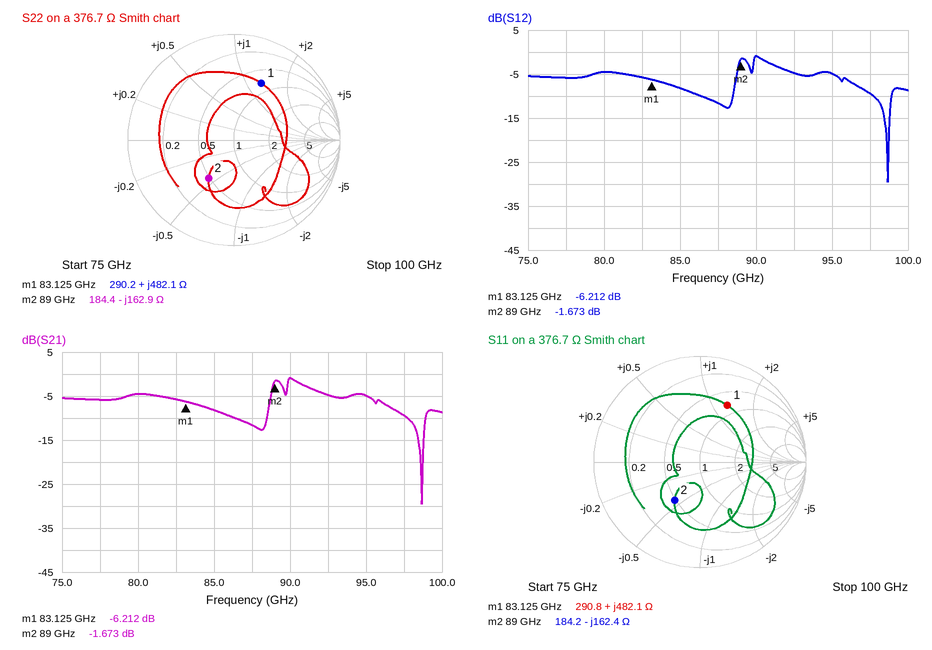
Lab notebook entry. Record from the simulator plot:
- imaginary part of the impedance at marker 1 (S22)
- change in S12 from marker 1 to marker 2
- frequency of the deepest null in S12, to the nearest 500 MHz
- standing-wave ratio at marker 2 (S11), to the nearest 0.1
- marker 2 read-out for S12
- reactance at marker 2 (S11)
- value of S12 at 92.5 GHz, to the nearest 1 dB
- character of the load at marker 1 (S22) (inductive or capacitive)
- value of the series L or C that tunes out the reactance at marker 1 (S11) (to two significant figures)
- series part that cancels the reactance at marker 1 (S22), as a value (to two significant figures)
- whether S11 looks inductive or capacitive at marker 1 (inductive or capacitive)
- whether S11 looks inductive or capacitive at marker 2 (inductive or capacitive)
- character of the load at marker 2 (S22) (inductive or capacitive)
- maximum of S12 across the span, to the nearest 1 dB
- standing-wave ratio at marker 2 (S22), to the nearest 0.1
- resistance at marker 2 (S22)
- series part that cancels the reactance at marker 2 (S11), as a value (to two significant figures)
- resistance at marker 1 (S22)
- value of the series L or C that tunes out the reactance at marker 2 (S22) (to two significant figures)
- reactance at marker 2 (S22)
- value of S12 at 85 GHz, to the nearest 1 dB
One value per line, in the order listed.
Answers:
+482.1 Ω
4.539 dB
98.5 GHz
2.5
-1.673 dB
-162.4 Ω
-5 dB
inductive
4.0 fF
4.0 fF
inductive
capacitive
capacitive
-1 dB
2.5
184.4 Ω
290 pH
290.2 Ω
290 pH
-162.9 Ω
-8 dB
